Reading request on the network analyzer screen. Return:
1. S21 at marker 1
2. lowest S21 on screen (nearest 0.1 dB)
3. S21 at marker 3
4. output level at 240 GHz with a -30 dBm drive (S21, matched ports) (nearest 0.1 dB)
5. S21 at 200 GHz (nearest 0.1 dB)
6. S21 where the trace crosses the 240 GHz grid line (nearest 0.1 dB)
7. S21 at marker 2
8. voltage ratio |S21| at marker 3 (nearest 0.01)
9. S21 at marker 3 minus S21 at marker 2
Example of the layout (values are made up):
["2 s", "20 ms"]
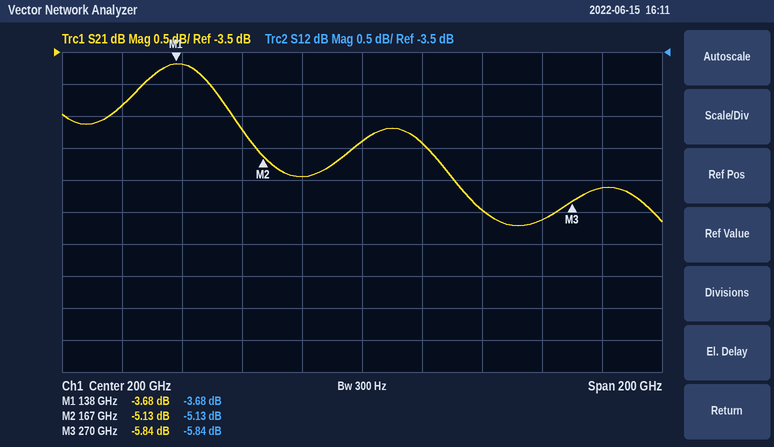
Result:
["-3.68 dB", "-6.2 dB", "-5.84 dB", "-36.0 dBm", "-4.9 dB", "-6.0 dB", "-5.13 dB", "0.51", "-0.71 dB"]
